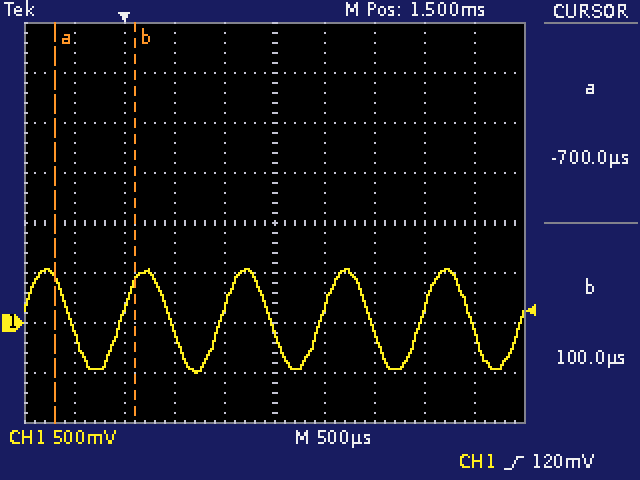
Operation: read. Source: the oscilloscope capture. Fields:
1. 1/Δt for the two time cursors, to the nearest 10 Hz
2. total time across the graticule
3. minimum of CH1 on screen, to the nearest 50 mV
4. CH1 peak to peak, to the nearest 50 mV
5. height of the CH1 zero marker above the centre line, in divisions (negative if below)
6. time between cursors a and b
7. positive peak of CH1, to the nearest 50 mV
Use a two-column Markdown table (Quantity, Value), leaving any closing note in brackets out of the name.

| Quantity | Value |
|---|---|
| 1/Δt for the two time cursors, to the nearest 10 Hz | 1.25 kHz |
| total time across the graticule | 5 ms |
| minimum of CH1 on screen, to the nearest 50 mV | -500 mV |
| CH1 peak to peak, to the nearest 50 mV | 1.05 V |
| height of the CH1 zero marker above the centre line, in divisions | -2.0 div |
| time between cursors a and b | 800 µs |
| positive peak of CH1, to the nearest 50 mV | 550 mV |
